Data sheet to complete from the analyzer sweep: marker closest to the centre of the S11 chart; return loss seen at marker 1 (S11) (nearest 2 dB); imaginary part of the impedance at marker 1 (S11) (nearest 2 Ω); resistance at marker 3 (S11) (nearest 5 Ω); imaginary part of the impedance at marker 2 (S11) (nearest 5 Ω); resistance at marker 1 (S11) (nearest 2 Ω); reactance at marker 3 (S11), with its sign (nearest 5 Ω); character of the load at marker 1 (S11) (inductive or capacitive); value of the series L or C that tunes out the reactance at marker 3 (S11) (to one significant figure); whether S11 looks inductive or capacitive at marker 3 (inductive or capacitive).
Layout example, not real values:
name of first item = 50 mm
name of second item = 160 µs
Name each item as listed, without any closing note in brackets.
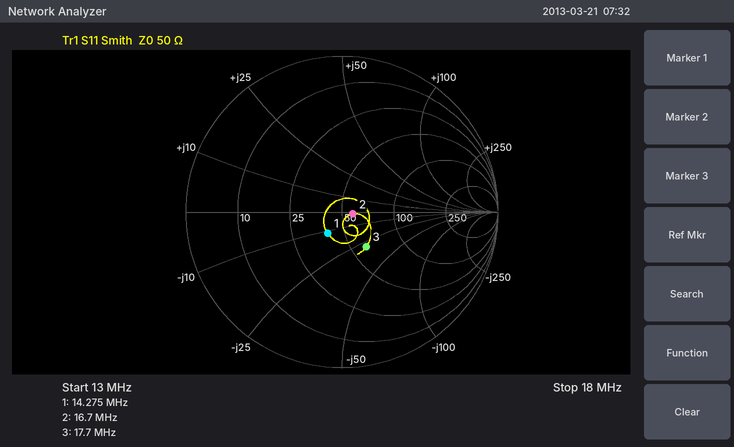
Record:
marker closest to the centre of the S11 chart = marker 2
return loss seen at marker 1 (S11) = 16 dB
imaginary part of the impedance at marker 1 (S11) = -12 Ω
resistance at marker 3 (S11) = 60 Ω
imaginary part of the impedance at marker 2 (S11) = 0 Ω
resistance at marker 1 (S11) = 40 Ω
reactance at marker 3 (S11), with its sign = -30 Ω
character of the load at marker 1 (S11) = capacitive
value of the series L or C that tunes out the reactance at marker 3 (S11) = 300 nH
whether S11 looks inductive or capacitive at marker 3 = capacitive
